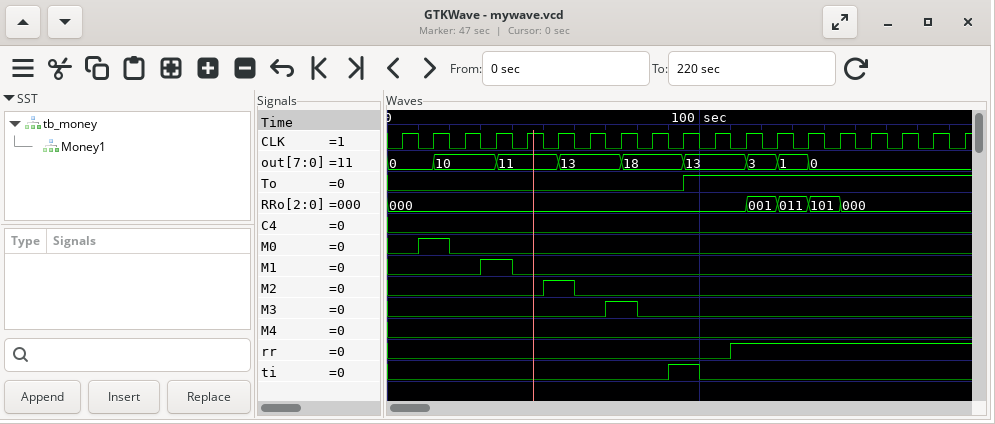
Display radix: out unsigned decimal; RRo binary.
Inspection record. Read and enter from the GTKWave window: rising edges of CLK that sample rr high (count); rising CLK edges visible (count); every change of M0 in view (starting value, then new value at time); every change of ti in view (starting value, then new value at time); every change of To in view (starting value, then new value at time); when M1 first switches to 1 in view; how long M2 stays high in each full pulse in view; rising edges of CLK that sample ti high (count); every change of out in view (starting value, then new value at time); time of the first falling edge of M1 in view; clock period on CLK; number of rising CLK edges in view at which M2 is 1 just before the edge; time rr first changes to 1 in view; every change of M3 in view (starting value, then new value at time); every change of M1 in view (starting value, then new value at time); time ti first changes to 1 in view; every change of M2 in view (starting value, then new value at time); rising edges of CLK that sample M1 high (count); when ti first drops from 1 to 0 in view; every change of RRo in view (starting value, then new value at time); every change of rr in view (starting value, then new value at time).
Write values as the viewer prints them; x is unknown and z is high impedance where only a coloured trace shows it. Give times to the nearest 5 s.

8
19
0, 1 at 10 s, 0 at 20 s
0, 1 at 90 s, 0 at 100 s
0, 1 at 95 s
30 s
10 s
1
0, 10 at 15 s, 11 at 35 s, 13 at 55 s, 18 at 75 s, 13 at 95 s, 3 at 115 s, 1 at 125 s, 0 at 135 s
40 s
10 s
1
110 s
0, 1 at 70 s, 0 at 80 s
0, 1 at 30 s, 0 at 40 s
90 s
0, 1 at 50 s, 0 at 60 s
1
100 s
000, 001 at 115 s, 011 at 125 s, 101 at 135 s, 000 at 145 s
0, 1 at 110 s
